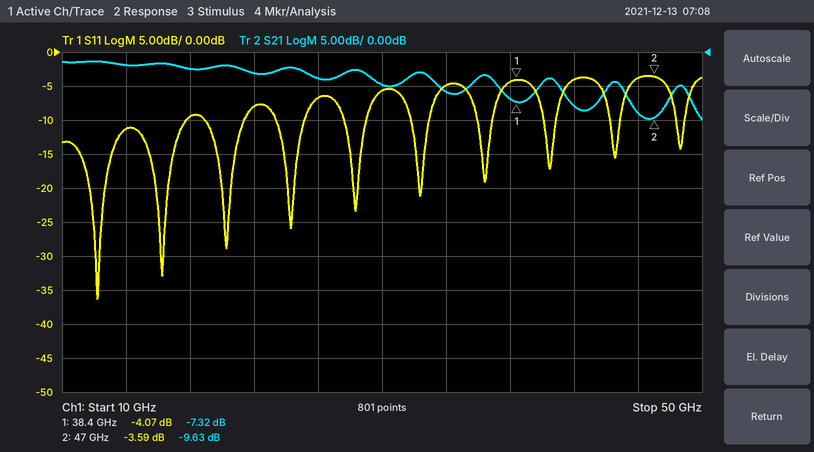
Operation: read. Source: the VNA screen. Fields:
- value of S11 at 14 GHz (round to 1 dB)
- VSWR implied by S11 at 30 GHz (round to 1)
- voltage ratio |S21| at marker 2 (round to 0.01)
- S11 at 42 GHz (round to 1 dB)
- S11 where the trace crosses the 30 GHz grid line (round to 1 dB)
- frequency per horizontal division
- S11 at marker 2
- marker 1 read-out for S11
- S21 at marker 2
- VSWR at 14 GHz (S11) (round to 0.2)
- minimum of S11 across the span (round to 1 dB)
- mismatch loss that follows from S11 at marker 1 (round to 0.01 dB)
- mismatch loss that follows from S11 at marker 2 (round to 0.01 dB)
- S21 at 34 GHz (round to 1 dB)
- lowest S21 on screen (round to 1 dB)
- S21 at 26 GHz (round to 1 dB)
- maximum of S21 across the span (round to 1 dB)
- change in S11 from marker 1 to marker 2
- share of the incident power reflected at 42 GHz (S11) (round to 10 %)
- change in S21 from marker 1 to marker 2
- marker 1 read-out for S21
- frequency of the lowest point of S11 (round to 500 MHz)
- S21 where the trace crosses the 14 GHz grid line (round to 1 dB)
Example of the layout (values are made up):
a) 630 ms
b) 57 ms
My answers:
a) -11 dB
b) 3
c) 0.33
d) -4 dB
e) -6 dB
f) 4 GHz
g) -3.59 dB
h) -4.07 dB
i) -9.63 dB
j) 1.8
k) -36 dB
l) 2.16 dB
m) 2.50 dB
n) -6 dB
o) -10 dB
p) -4 dB
q) -1 dB
r) 0.48 dB
s) 40 %
t) -2.31 dB
u) -7.32 dB
v) 12.0 GHz
w) -2 dB
